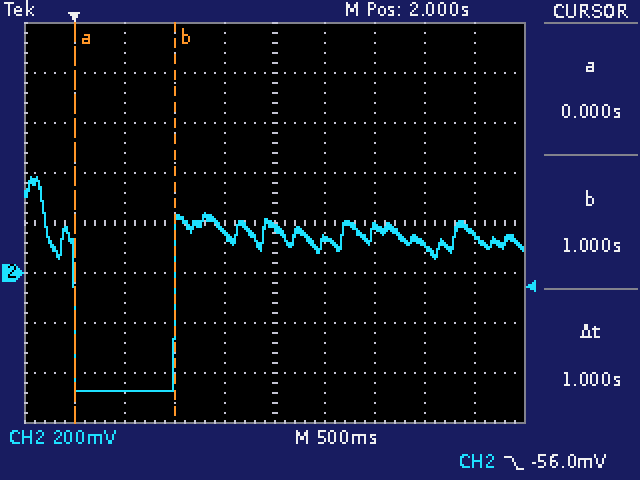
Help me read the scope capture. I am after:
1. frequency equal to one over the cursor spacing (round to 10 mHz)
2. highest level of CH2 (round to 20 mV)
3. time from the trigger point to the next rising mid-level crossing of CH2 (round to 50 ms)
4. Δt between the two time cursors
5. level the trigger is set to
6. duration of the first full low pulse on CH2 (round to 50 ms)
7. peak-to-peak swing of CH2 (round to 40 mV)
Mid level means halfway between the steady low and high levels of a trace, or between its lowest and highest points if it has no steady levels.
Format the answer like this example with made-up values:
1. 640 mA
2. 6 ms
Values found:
1. 1.00 Hz
2. 380 mV
3. 1.00 s
4. 1 s
5. -56.0 mV
6. 1.00 s
7. 840 mV
